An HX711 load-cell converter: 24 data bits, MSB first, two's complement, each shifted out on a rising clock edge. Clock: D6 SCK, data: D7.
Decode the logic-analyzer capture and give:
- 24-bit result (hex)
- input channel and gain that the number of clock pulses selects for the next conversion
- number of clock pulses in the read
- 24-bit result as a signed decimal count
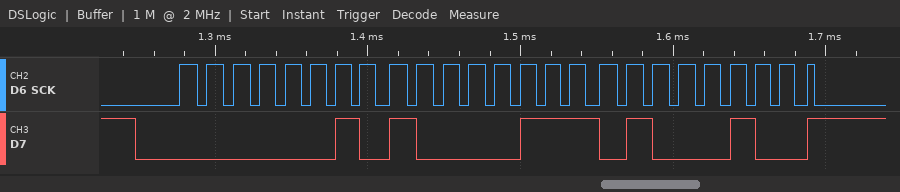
0x028744
channel A, gain 128
25
165700
